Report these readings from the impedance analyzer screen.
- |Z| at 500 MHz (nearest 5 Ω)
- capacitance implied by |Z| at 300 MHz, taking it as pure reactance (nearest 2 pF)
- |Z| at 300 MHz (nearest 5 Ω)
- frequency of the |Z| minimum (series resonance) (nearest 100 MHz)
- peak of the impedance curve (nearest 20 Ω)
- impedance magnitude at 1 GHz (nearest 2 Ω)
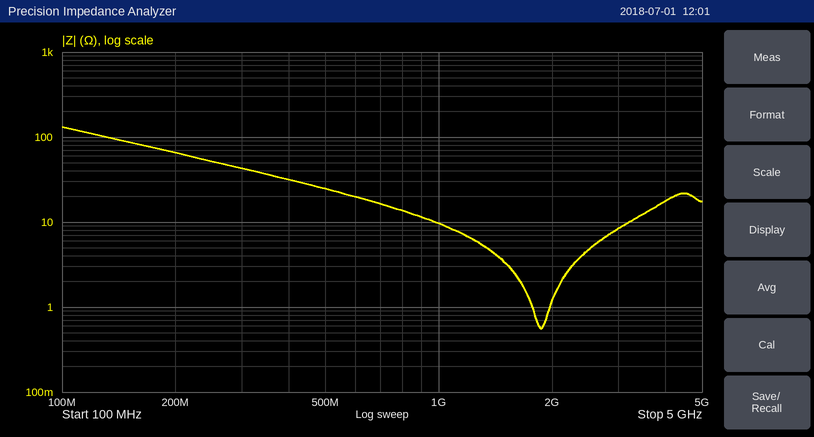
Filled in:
25 Ω
12 pF
45 Ω
1.9 GHz
140 Ω
10 Ω
